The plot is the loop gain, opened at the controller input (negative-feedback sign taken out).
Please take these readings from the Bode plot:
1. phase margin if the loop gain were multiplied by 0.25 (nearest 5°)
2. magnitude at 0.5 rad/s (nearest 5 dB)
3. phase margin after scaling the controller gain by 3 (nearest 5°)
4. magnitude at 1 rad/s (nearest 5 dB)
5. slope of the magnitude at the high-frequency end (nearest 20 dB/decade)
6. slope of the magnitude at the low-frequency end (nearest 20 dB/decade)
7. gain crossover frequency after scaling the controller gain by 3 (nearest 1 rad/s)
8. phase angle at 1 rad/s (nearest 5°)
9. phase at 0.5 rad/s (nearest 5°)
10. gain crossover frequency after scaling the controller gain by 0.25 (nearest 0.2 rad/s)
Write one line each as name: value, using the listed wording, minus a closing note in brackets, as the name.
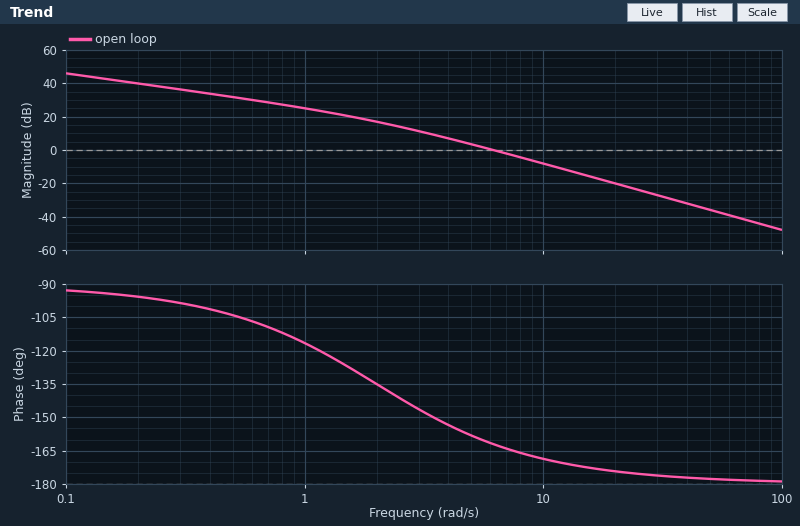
phase margin if the loop gain were multiplied by 0.25: 35°
magnitude at 0.5 rad/s: 30 dB
phase margin after scaling the controller gain by 3: 10°
magnitude at 1 rad/s: 25 dB
slope of the magnitude at the high-frequency end: -40 dB/decade
slope of the magnitude at the low-frequency end: -20 dB/decade
gain crossover frequency after scaling the controller gain by 3: 11 rad/s
phase angle at 1 rad/s: -115°
phase at 0.5 rad/s: -105°
gain crossover frequency after scaling the controller gain by 0.25: 2.8 rad/s
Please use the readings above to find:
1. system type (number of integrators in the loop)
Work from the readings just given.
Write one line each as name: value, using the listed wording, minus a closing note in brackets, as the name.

system type: 1
